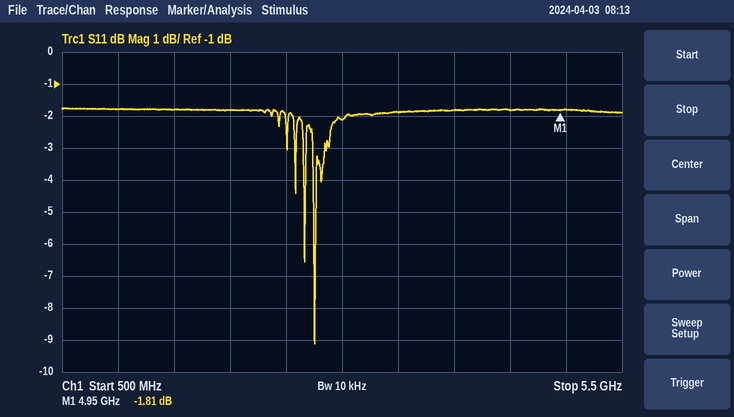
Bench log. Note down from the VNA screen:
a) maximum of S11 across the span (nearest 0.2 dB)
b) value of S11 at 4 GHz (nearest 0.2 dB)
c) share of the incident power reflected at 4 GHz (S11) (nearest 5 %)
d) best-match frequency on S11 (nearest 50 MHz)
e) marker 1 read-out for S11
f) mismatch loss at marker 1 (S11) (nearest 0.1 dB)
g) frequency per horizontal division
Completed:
-1.8 dB
-1.8 dB
65 %
2.75 GHz
-1.81 dB
4.7 dB
500 MHz
